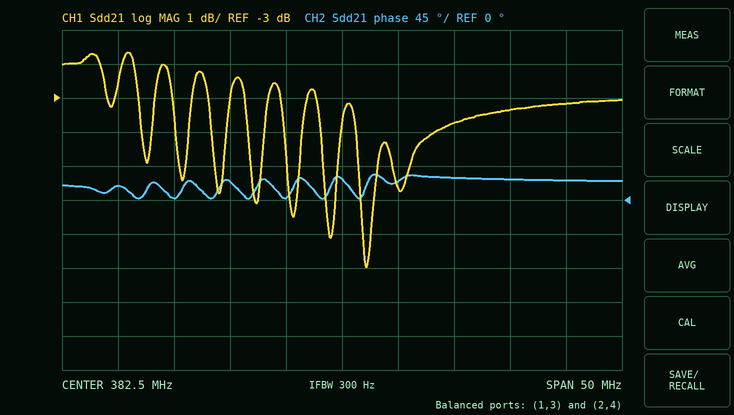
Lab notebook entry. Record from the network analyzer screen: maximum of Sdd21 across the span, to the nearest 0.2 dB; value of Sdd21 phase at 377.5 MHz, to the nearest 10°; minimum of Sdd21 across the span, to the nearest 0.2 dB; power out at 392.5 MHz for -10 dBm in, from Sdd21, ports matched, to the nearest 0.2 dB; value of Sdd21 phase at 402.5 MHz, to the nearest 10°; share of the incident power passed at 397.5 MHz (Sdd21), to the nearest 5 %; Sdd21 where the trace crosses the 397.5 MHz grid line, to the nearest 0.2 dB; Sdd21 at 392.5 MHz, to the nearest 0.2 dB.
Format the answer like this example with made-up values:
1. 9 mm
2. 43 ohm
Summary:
1. -1.6 dB
2. 0°
3. -8.0 dB
4. -13.8 dBm
5. 30°
6. 45 %
7. -3.4 dB
8. -3.8 dB
